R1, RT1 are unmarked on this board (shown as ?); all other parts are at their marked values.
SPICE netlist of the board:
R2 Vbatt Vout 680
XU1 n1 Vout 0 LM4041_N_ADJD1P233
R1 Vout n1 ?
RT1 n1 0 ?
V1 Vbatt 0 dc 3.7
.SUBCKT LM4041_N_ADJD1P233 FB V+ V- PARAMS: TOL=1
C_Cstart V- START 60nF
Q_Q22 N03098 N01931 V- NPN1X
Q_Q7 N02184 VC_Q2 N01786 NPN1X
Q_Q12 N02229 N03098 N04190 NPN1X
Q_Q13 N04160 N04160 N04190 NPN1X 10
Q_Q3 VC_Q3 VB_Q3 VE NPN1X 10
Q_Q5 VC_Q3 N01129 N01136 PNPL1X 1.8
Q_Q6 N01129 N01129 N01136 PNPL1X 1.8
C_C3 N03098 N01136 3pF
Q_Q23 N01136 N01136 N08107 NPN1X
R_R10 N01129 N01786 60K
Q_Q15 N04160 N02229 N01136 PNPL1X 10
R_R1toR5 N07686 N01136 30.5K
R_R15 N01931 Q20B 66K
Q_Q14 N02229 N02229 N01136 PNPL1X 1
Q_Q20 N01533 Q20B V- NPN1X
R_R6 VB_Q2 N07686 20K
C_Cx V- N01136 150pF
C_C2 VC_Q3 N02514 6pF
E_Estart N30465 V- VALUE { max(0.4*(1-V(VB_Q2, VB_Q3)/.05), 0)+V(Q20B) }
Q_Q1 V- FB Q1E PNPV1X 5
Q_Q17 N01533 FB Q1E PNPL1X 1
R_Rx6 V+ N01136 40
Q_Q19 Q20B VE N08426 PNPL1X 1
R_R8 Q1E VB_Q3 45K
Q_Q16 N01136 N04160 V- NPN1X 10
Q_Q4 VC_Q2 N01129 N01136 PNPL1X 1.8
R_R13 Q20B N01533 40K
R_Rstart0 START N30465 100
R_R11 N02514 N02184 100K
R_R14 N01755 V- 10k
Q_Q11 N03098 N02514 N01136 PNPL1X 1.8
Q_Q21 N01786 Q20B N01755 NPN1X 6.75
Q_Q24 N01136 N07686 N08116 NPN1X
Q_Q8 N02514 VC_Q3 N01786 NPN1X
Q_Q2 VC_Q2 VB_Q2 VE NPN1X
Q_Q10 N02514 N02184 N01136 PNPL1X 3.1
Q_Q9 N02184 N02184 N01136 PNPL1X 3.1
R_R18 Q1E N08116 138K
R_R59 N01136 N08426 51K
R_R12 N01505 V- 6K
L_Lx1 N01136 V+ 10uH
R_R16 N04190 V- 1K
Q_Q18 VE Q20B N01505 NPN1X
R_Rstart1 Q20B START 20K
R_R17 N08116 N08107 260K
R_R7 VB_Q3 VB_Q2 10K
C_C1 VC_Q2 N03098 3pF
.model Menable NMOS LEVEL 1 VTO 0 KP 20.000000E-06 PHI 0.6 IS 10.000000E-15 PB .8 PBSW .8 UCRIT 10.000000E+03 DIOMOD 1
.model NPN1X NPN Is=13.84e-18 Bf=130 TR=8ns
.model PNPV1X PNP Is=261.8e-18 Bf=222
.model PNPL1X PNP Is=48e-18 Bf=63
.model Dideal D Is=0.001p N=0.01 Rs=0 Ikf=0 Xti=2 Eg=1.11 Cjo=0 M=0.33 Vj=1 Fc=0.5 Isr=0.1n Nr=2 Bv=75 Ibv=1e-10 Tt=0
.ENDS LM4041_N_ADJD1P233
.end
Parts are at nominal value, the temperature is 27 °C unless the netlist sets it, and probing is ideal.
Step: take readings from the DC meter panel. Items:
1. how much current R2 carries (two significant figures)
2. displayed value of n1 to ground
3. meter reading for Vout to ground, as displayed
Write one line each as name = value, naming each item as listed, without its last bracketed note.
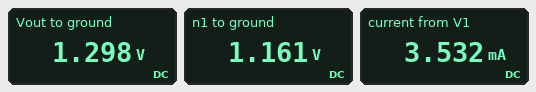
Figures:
how much current R2 carries = 3.5 mA
displayed value of n1 to ground = 1.161 V
meter reading for Vout to ground, as displayed = 1.298 V
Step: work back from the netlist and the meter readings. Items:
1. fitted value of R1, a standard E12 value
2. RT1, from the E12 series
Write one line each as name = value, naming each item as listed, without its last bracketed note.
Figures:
fitted value of R1, a standard E12 value = 39 Ω
RT1, from the E12 series = 330 Ω
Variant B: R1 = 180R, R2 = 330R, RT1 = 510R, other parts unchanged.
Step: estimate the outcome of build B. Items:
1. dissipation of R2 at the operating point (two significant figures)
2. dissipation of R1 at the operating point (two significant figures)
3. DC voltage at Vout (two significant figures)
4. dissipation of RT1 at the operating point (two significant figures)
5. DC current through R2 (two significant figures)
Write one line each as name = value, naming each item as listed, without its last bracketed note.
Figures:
dissipation of R2 at the operating point = 4.4 mW
dissipation of R1 at the operating point = 2.4 mW
DC voltage at Vout = 2.5 V
dissipation of RT1 at the operating point = 6.7 mW
DC current through R2 = 3.6 mA
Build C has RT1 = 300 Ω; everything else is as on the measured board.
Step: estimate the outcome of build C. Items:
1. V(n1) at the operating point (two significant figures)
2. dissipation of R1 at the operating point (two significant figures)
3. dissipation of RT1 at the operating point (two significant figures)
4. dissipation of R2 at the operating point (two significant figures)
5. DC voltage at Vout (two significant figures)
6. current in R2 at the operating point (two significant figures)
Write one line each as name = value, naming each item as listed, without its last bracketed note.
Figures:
V(n1) at the operating point = 1.1 V
dissipation of R1 at the operating point = 510 µW
dissipation of RT1 at the operating point = 3.9 mW
dissipation of R2 at the operating point = 9.0 mW
DC voltage at Vout = 1.2 V
current in R2 at the operating point = 3.6 mA
